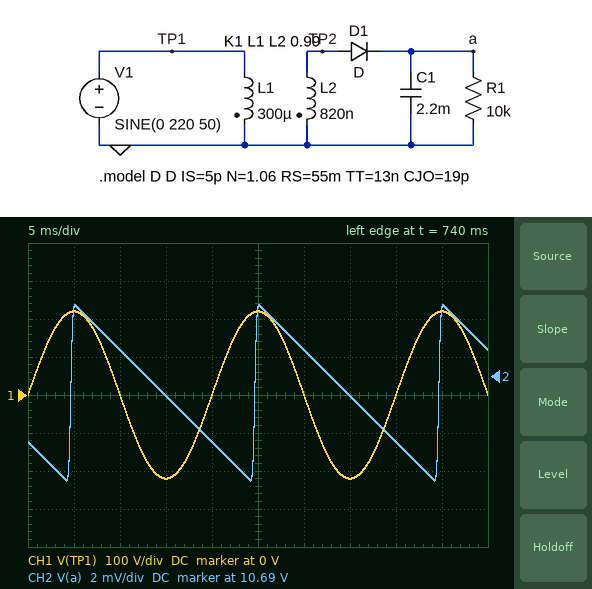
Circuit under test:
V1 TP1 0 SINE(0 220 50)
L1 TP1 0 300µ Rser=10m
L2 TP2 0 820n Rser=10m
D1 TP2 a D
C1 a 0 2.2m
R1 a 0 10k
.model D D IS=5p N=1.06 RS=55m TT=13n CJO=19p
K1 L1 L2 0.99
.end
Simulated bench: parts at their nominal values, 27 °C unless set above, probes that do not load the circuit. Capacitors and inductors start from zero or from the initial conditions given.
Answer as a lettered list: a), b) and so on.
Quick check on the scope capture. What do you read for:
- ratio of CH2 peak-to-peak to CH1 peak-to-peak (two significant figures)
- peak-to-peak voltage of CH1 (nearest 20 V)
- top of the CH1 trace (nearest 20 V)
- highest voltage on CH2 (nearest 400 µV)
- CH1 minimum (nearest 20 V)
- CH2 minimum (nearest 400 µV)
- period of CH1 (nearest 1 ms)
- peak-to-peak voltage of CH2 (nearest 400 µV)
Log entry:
a) 0.000021
b) 440 V
c) 220 V
d) 10.6916 V
e) -220 V
f) 10.6824 V
g) 20 ms
h) 9.2 mV
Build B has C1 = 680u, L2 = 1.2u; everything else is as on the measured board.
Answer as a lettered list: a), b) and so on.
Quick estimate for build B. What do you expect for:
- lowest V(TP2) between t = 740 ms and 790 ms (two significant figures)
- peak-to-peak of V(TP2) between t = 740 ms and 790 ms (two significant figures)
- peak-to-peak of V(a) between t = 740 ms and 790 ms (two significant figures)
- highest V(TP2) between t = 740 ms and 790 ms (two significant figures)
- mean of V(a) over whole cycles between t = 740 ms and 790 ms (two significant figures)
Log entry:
a) -14 V
b) 27 V
c) 37 mV
d) 14 V
e) 13 V
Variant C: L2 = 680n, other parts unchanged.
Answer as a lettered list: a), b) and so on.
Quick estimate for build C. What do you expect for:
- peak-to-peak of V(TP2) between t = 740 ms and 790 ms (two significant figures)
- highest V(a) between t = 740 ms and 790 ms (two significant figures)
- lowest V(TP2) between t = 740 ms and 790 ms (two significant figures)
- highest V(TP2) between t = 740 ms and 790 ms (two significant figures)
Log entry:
a) 21 V
b) 9.7 V
c) -10 V
d) 10 V
